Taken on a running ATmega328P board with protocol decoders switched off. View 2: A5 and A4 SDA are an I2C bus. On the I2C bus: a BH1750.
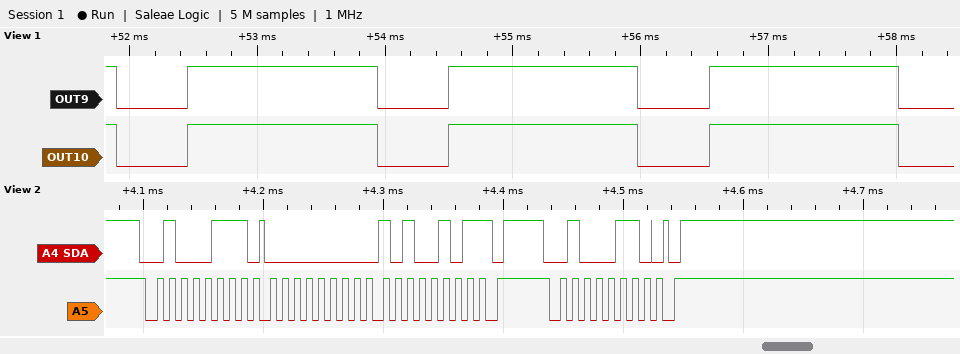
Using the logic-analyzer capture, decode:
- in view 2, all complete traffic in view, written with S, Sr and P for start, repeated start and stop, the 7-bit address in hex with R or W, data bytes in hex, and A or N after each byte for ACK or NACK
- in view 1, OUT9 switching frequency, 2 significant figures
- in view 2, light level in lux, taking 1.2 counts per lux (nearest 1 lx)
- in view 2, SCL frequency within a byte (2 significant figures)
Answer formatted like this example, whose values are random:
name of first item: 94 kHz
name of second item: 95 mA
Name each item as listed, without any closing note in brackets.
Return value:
in view 2, all complete traffic in view, written with S, Sr and P for start, repeated start and stop, the 7-bit address in hex with R or W, data bytes in hex, and A or N after each byte for ACK or NACK: S 23R A 00 A A5 N P S 23W A P
in view 1, OUT9 switching frequency, 2 significant figures: 490 Hz
in view 2, light level in lux, taking 1.2 counts per lux: 138 lx
in view 2, SCL frequency within a byte: 100 kHz
